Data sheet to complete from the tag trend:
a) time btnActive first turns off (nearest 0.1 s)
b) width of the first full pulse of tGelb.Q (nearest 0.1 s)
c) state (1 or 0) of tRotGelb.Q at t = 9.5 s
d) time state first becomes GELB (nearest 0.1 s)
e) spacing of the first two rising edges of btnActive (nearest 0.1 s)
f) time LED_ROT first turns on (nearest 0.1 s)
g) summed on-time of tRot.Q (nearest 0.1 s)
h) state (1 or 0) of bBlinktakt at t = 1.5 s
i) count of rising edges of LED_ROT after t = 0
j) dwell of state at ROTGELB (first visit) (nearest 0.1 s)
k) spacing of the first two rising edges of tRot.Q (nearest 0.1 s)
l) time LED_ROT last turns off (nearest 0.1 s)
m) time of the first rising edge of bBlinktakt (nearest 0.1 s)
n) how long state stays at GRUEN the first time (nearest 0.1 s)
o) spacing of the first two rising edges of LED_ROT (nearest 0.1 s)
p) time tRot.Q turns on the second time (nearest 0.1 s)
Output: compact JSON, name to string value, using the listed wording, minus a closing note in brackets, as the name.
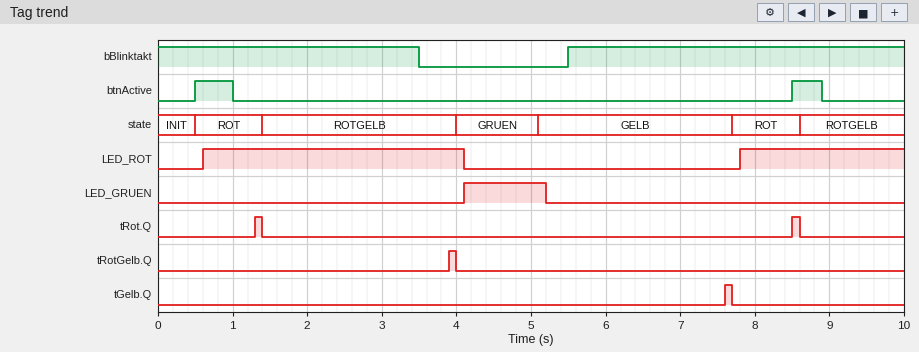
{"time btnActive first turns off": "1.0 s", "width of the first full pulse of tGelb.Q": "0.1 s", "state (1 or 0) of tRotGelb.Q at t = 9.5 s": "0", "time state first becomes GELB": "5.1 s", "spacing of the first two rising edges of btnActive": "8.0 s", "time LED_ROT first turns on": "0.6 s", "summed on-time of tRot.Q": "0.2 s", "state (1 or 0) of bBlinktakt at t = 1.5 s": "1", "count of rising edges of LED_ROT after t = 0": "2", "dwell of state at ROTGELB (first visit)": "2.6 s", "spacing of the first two rising edges of tRot.Q": "7.2 s", "time LED_ROT last turns off": "4.1 s", "time of the first rising edge of bBlinktakt": "5.5 s", "how long state stays at GRUEN the first time": "1.1 s", "spacing of the first two rising edges of LED_ROT": "7.2 s", "time tRot.Q turns on the second time": "8.5 s"}
